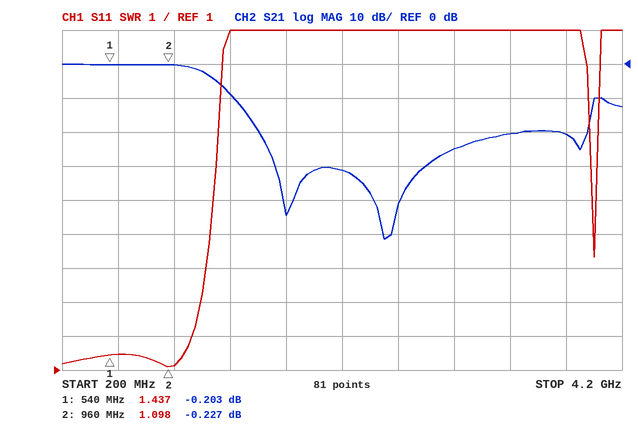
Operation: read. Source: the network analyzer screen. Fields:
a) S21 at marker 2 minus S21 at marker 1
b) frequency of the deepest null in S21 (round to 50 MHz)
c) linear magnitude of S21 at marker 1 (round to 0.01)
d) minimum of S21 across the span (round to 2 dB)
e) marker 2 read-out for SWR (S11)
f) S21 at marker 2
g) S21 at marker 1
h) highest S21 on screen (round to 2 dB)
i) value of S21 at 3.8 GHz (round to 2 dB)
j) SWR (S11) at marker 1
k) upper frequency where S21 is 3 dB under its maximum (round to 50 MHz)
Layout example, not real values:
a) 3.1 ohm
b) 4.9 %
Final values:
a) -0.024 dB
b) 2.50 GHz
c) 0.98
d) -52 dB
e) 1.098
f) -0.227 dB
g) -0.203 dB
h) 0 dB
i) -20 dB
j) 1.437
k) 1.25 GHz
